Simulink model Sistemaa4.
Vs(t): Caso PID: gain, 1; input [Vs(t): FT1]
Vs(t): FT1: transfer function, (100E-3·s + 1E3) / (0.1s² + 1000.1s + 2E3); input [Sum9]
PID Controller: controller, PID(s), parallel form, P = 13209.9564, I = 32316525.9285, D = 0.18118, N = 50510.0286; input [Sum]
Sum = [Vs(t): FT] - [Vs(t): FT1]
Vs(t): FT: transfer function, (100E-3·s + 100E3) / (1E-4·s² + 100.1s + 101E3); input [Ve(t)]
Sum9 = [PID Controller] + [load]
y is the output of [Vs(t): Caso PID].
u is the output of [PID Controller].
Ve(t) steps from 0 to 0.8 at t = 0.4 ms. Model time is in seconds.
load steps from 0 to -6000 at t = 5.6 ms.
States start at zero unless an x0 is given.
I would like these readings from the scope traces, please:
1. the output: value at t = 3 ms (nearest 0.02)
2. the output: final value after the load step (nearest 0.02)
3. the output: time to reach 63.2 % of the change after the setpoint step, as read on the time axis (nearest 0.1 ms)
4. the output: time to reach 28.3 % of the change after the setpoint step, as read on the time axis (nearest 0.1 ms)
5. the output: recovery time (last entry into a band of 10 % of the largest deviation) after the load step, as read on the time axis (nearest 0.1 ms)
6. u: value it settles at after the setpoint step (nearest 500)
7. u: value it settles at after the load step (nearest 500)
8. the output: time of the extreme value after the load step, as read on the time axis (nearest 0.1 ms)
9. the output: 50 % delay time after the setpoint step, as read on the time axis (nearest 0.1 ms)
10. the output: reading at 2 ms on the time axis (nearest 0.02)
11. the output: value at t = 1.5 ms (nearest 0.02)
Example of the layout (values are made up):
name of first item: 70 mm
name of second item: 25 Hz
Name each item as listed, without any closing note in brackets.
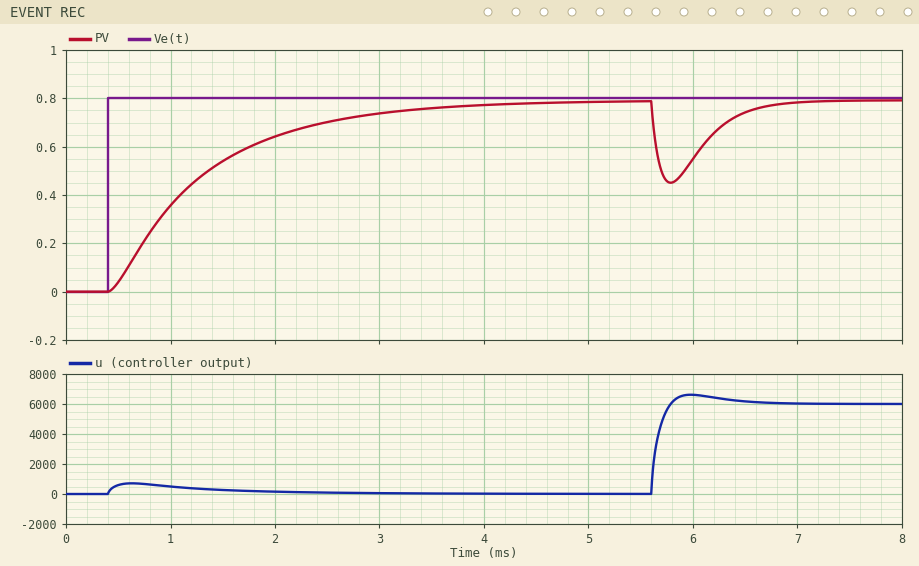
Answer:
the output: value at t = 3 ms: 0.74
the output: final value after the load step: 0.80
the output: time to reach 63.2 % of the change after the setpoint step, as read on the time axis: 1.4 ms
the output: time to reach 28.3 % of the change after the setpoint step, as read on the time axis: 0.8 ms
the output: recovery time (last entry into a band of 10 % of the largest deviation) after the load step, as read on the time axis: 6.6 ms
u: value it settles at after the setpoint step: 0
u: value it settles at after the load step: 6000
the output: time of the extreme value after the load step, as read on the time axis: 5.8 ms
the output: 50 % delay time after the setpoint step, as read on the time axis: 1.1 ms
the output: reading at 2 ms on the time axis: 0.64
the output: value at t = 1.5 ms: 0.54
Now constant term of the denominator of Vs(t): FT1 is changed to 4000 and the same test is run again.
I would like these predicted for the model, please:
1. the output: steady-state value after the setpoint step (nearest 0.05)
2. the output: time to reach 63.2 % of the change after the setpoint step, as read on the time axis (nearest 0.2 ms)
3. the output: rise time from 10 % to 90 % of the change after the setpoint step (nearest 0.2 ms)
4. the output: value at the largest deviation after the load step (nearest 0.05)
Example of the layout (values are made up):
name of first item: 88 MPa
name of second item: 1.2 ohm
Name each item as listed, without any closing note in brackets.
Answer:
the output: steady-state value after the setpoint step: 0.80
the output: time to reach 63.2 % of the change after the setpoint step, as read on the time axis: 1.4 ms
the output: rise time from 10 % to 90 % of the change after the setpoint step: 2.0 ms
the output: value at the largest deviation after the load step: 0.45
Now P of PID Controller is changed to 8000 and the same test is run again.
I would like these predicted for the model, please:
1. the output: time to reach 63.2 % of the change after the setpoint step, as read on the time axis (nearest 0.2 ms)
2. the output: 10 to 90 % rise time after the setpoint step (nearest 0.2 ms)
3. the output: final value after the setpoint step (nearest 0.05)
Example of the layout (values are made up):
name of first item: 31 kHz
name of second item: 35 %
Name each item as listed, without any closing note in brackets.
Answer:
the output: time to reach 63.2 % of the change after the setpoint step, as read on the time axis: 1.4 ms
the output: 10 to 90 % rise time after the setpoint step: 2.0 ms
the output: final value after the setpoint step: 0.80
